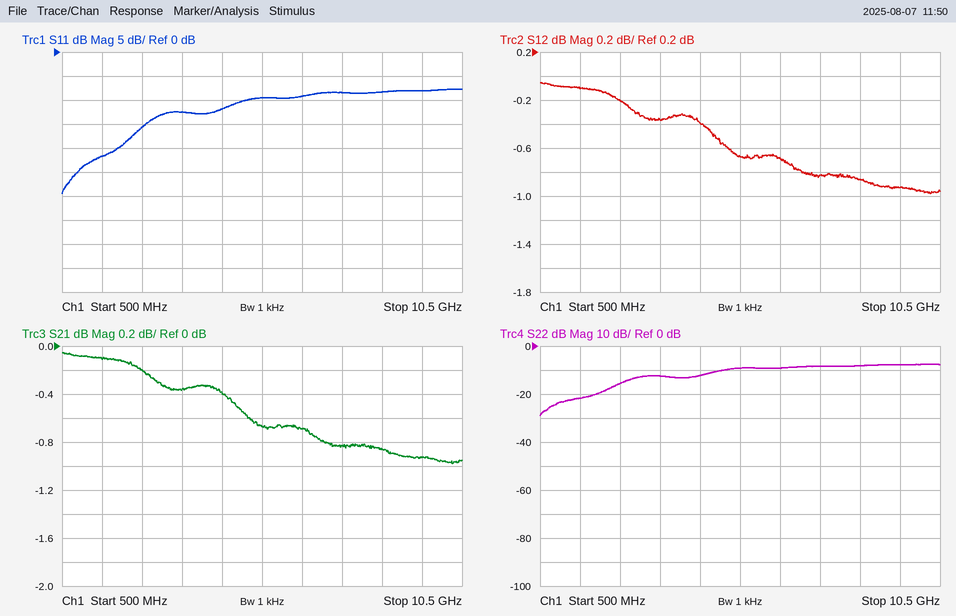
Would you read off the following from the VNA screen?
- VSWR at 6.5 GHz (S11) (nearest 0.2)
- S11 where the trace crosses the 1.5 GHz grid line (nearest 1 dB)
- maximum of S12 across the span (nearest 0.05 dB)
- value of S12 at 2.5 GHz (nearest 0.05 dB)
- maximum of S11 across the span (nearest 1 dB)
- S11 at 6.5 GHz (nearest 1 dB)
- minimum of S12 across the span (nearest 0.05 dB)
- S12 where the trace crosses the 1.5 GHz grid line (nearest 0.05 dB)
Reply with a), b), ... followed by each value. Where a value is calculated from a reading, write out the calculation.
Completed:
a) |Γ| = 10^(-9/20) = 0.3548; VSWR = (1 + 0.3548)/(1 − 0.3548) ≈ 2.10, so 2.0 to the nearest 0.2
b) -22 dB
c) -0.05 dB
d) -0.20 dB
e) -8 dB
f) -9 dB
g) -1.00 dB
h) -0.10 dB
